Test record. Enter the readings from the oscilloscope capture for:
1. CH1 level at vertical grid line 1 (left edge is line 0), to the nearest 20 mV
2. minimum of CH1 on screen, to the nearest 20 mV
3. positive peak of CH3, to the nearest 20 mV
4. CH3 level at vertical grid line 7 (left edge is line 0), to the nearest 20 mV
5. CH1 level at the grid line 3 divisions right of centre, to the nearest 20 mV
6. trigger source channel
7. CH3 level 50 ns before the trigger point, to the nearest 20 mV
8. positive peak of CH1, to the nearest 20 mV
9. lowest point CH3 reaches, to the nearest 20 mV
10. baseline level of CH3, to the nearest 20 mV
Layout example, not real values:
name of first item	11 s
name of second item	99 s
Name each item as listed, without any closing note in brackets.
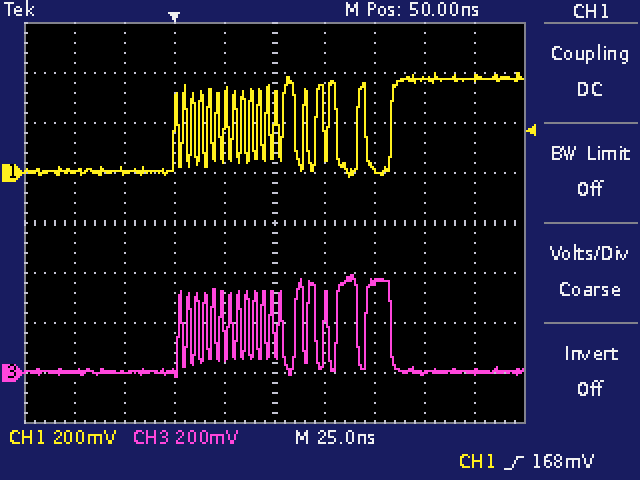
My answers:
CH1 level at vertical grid line 1 (left edge is line 0), to the nearest 20 mV	0 mV
minimum of CH1 on screen, to the nearest 20 mV	-20 mV
positive peak of CH3, to the nearest 20 mV	400 mV
CH3 level at vertical grid line 7 (left edge is line 0), to the nearest 20 mV	360 mV
CH1 level at the grid line 3 divisions right of centre, to the nearest 20 mV	380 mV
trigger source channel	CH1
CH3 level 50 ns before the trigger point, to the nearest 20 mV	0 mV
positive peak of CH1, to the nearest 20 mV	400 mV
lowest point CH3 reaches, to the nearest 20 mV	-20 mV
baseline level of CH3, to the nearest 20 mV	0 mV
